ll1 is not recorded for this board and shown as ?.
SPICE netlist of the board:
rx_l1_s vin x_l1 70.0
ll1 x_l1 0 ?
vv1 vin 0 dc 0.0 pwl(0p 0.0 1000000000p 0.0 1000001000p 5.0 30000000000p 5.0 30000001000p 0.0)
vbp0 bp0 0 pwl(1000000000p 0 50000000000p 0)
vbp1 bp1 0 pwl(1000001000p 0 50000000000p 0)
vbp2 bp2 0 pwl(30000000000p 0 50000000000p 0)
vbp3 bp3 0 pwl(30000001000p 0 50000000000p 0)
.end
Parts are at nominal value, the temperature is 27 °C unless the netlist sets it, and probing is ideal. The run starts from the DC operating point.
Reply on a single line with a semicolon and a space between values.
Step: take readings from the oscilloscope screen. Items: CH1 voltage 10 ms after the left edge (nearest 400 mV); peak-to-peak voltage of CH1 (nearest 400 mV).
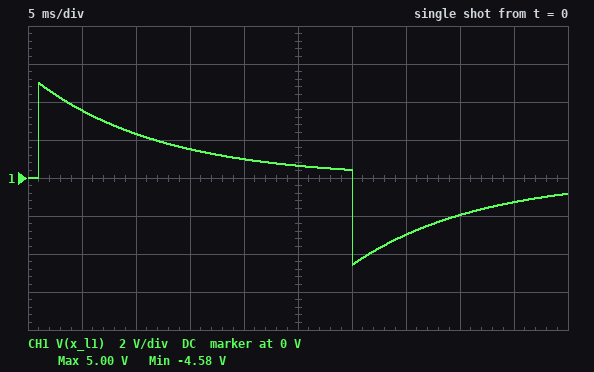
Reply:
2.4 V; 9.6 V
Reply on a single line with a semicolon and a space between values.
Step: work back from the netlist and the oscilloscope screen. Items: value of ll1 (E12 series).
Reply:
820 mH
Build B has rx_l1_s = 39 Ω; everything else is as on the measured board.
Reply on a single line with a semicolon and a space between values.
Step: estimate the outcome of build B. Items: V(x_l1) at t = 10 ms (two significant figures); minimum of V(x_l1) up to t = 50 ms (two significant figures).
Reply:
3.3 V; -3.7 V
